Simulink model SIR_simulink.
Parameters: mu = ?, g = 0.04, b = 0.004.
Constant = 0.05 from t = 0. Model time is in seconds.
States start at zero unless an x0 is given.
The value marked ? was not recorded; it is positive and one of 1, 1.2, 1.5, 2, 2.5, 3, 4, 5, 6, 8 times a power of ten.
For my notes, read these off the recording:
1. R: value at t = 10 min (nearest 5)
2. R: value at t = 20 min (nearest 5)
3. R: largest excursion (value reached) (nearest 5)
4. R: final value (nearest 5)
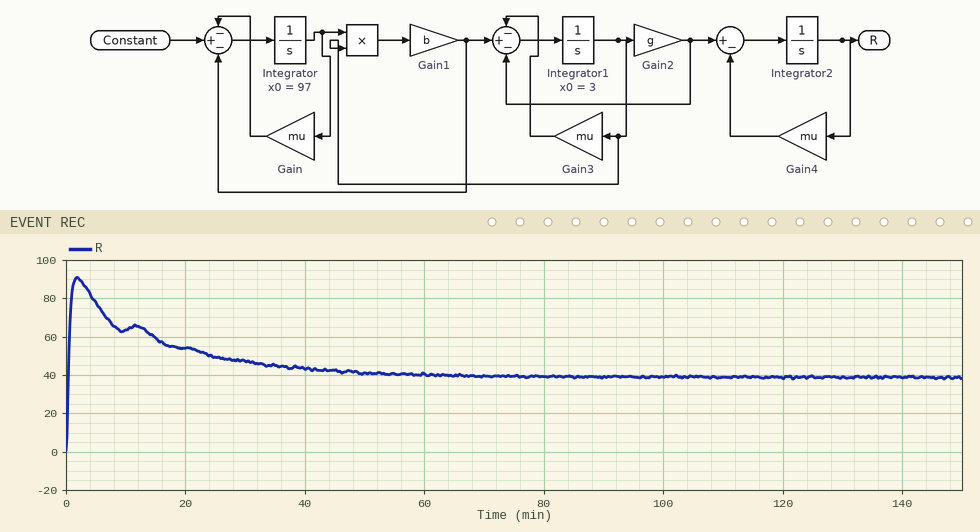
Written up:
65
55
90
40
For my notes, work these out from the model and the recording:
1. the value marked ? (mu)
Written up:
0.001
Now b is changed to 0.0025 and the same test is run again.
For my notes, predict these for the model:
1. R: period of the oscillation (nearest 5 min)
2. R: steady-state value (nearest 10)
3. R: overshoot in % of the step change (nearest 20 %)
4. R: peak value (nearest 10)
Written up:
15 min
30
180 %
90
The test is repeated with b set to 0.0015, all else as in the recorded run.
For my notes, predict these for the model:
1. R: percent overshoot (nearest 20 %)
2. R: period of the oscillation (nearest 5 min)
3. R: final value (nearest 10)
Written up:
280 %
30 min
20
